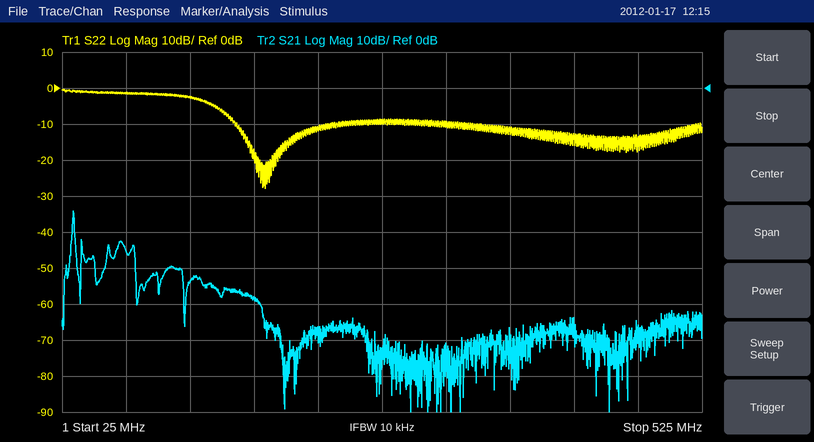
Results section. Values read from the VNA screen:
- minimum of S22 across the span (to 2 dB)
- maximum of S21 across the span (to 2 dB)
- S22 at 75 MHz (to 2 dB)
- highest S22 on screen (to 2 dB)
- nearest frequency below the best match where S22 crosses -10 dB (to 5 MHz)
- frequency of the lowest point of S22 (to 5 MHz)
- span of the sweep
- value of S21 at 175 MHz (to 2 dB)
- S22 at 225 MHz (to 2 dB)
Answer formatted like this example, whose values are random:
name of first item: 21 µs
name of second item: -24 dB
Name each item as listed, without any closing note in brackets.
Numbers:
minimum of S22 across the span: -28 dB
maximum of S21 across the span: -34 dB
S22 at 75 MHz: -2 dB
highest S22 on screen: 0 dB
nearest frequency below the best match where S22 crosses -10 dB: 160 MHz
frequency of the lowest point of S22: 185 MHz
span of the sweep: 500 MHz
value of S21 at 175 MHz: -58 dB
S22 at 225 MHz: -12 dB
